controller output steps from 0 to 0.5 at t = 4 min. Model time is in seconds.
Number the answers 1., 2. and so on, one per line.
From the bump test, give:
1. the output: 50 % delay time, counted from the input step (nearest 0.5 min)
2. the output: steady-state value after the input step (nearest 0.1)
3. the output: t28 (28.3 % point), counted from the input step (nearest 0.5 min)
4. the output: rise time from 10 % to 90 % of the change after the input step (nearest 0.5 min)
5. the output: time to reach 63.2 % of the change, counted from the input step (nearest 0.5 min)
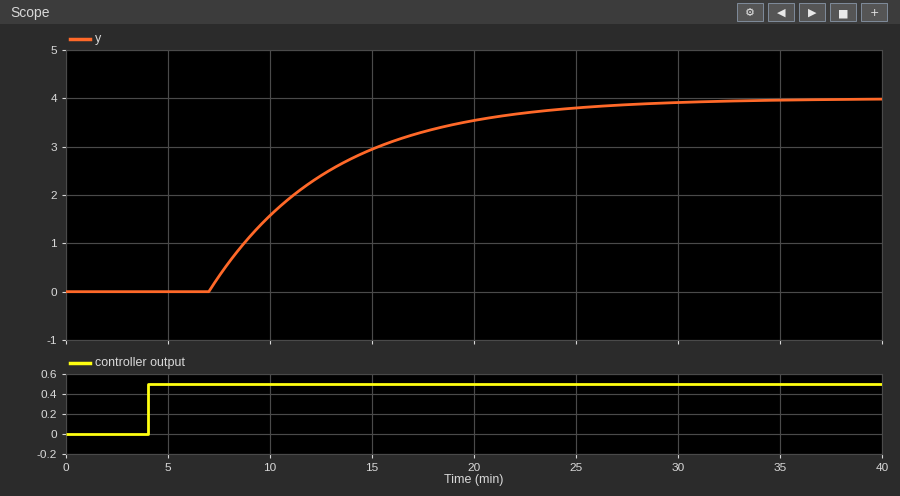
1. 7.0 min
2. 4.0
3. 5.0 min
4. 13.0 min
5. 9.0 min
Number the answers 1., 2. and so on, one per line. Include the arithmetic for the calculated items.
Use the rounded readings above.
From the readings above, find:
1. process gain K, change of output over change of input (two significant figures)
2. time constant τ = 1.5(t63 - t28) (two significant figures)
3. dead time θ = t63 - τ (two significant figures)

1. (4 - 0) / 0.5 = 8.0
2. 1.5 × (9 - 5) = 6.0 min
3. 9 - 6 = 3.0 min
